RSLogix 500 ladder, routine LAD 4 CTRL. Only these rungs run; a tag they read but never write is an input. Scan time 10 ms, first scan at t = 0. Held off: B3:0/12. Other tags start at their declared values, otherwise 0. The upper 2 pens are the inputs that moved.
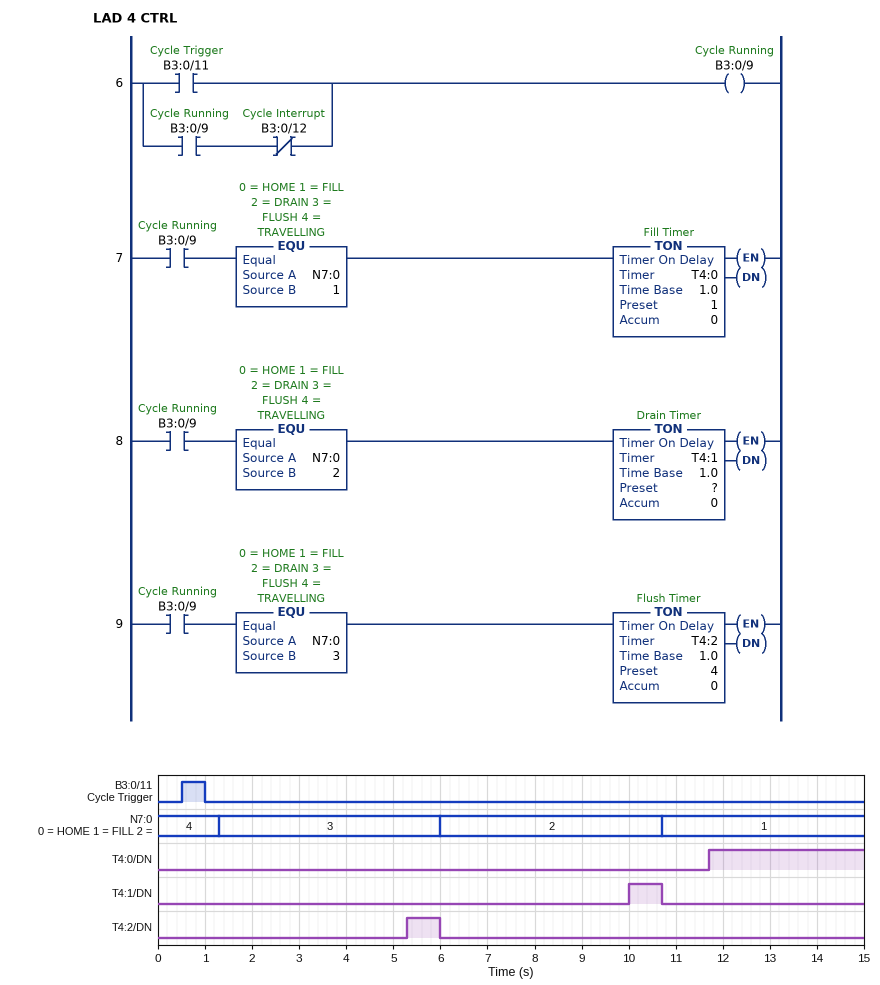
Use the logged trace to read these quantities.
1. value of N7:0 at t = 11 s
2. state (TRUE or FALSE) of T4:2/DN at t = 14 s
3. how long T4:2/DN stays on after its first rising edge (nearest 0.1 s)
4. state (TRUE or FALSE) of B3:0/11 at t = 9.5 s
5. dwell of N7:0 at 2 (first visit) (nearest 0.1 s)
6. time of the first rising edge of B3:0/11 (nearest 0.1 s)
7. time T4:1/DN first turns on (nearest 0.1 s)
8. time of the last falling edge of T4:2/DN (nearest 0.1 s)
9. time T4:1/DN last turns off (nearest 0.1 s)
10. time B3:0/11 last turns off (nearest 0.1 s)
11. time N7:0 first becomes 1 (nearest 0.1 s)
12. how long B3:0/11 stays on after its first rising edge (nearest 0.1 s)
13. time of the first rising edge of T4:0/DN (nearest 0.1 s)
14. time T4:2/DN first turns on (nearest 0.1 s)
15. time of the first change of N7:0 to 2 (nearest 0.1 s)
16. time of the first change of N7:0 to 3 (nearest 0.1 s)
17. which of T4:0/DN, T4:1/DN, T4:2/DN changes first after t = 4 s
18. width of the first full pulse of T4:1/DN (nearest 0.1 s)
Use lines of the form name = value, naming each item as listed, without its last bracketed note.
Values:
value of N7:0 at t = 11 s = 1
state (TRUE or FALSE) of T4:2/DN at t = 14 s = FALSE
how long T4:2/DN stays on after its first rising edge = 0.7 s
state (TRUE or FALSE) of B3:0/11 at t = 9.5 s = FALSE
dwell of N7:0 at 2 (first visit) = 4.7 s
time of the first rising edge of B3:0/11 = 0.5 s
time T4:1/DN first turns on = 10.0 s
time of the last falling edge of T4:2/DN = 6.0 s
time T4:1/DN last turns off = 10.7 s
time B3:0/11 last turns off = 1.0 s
time N7:0 first becomes 1 = 10.7 s
how long B3:0/11 stays on after its first rising edge = 0.5 s
time of the first rising edge of T4:0/DN = 11.7 s
time T4:2/DN first turns on = 5.3 s
time of the first change of N7:0 to 2 = 6.0 s
time of the first change of N7:0 to 3 = 1.3 s
which of T4:0/DN, T4:1/DN, T4:2/DN changes first after t = 4 s = T4:2/DN
width of the first full pulse of T4:1/DN = 0.7 s
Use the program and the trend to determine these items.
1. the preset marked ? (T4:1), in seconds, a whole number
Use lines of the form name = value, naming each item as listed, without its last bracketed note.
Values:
the preset marked ? (T4:1), in seconds, a whole number = 4 s
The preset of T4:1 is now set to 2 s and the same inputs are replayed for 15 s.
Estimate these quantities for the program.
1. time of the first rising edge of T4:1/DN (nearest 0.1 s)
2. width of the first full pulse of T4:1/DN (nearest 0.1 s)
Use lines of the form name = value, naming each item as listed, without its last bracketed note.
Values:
time of the first rising edge of T4:1/DN = 8.0 s
width of the first full pulse of T4:1/DN = 2.7 s
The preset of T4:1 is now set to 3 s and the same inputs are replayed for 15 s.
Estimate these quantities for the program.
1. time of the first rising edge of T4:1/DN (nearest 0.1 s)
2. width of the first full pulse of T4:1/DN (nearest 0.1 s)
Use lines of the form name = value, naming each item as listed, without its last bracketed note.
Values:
time of the first rising edge of T4:1/DN = 9.0 s
width of the first full pulse of T4:1/DN = 1.7 s
